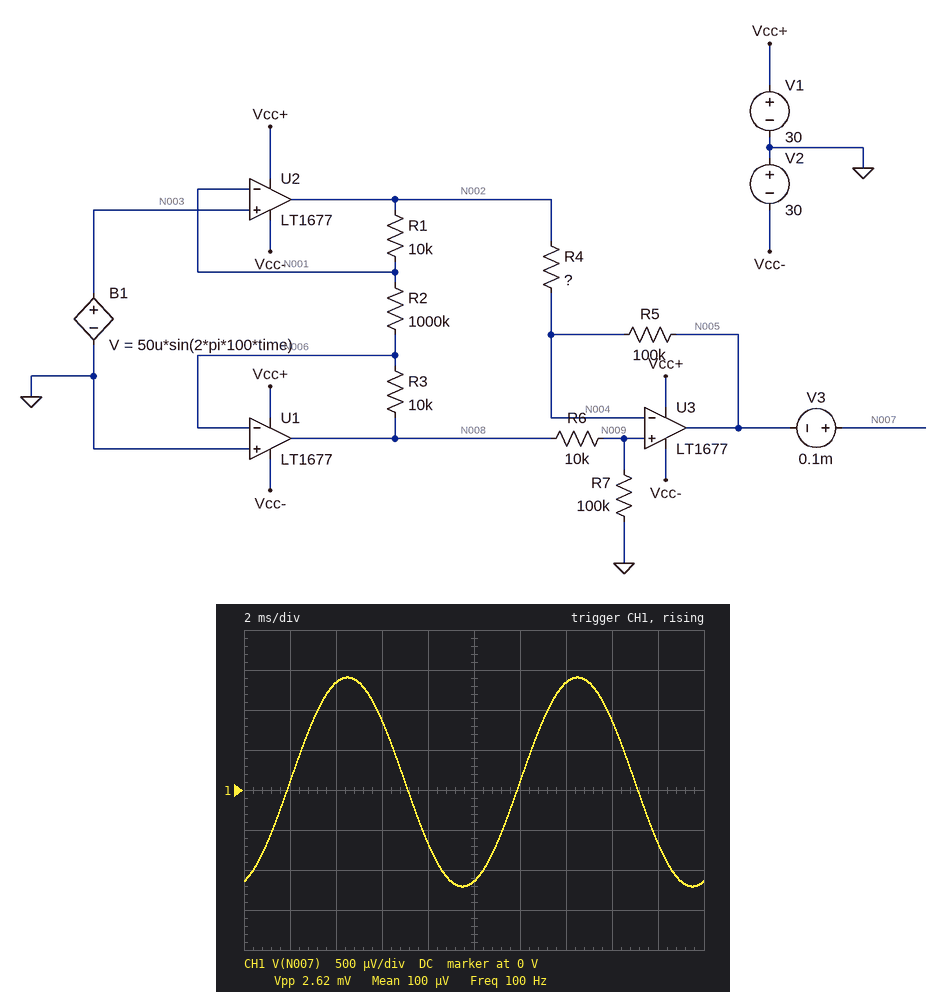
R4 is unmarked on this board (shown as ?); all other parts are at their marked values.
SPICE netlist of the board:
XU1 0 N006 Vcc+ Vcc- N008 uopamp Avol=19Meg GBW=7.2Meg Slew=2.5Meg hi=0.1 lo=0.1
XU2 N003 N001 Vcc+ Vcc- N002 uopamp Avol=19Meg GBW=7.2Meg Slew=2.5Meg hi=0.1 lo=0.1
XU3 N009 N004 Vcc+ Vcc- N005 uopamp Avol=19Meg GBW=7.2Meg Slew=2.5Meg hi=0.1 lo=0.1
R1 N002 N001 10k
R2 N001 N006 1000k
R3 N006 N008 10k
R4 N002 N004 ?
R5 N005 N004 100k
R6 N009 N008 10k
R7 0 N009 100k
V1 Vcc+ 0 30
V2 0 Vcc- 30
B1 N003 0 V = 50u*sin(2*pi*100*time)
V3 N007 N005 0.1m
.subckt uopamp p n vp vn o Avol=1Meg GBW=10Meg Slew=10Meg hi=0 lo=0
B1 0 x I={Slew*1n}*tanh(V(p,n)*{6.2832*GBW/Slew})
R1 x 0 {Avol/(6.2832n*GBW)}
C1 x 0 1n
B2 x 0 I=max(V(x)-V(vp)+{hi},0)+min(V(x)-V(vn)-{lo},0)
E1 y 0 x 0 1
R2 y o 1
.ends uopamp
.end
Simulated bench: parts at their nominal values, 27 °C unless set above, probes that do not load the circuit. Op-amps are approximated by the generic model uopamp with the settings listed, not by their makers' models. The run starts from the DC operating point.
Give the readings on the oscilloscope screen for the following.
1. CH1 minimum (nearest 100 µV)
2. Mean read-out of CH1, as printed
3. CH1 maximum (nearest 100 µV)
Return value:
-1.2 mV
100 µV
1.4 mV
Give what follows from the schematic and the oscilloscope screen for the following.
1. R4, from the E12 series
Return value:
3.9 kΩ
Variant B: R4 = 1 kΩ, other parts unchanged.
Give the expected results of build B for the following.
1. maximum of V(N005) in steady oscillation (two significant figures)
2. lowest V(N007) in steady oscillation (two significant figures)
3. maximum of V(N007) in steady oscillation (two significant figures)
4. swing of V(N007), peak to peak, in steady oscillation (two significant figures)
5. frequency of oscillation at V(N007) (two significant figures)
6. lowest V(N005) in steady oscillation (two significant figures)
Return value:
5.1 mV
-5.0 mV
5.2 mV
10 mV
100 Hz
-5.1 mV
